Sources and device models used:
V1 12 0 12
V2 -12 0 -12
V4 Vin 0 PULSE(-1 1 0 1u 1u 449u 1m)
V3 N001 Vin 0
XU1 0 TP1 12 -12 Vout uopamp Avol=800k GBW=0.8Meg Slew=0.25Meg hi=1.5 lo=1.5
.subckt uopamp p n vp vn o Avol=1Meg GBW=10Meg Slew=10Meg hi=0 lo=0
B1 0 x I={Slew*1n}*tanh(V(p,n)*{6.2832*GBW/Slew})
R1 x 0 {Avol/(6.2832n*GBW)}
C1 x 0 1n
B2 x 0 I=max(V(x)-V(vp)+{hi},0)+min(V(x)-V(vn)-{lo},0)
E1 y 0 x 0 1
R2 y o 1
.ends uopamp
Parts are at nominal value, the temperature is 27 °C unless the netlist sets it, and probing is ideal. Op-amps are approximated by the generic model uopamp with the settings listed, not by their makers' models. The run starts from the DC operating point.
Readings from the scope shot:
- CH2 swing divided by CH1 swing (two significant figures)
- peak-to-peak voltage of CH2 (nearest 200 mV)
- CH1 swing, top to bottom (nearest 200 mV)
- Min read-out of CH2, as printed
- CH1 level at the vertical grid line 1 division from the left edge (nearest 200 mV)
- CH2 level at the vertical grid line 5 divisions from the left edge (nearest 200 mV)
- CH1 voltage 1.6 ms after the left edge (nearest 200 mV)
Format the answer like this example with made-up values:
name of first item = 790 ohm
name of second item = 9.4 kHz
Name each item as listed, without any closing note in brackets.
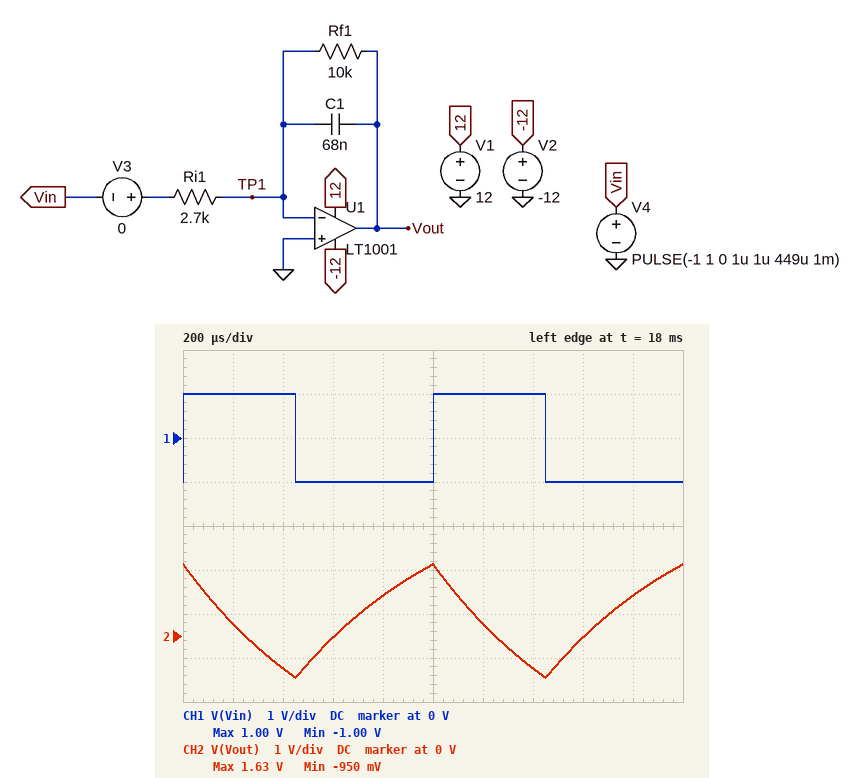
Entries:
CH2 swing divided by CH1 swing = 1.3
peak-to-peak voltage of CH2 = 2.6 V
CH1 swing, top to bottom = 2.0 V
Min read-out of CH2, as printed = -950 mV
CH1 level at the vertical grid line 1 division from the left edge = 1.0 V
CH2 level at the vertical grid line 5 divisions from the left edge = 1.6 V
CH1 voltage 1.6 ms after the left edge = -1.0 V
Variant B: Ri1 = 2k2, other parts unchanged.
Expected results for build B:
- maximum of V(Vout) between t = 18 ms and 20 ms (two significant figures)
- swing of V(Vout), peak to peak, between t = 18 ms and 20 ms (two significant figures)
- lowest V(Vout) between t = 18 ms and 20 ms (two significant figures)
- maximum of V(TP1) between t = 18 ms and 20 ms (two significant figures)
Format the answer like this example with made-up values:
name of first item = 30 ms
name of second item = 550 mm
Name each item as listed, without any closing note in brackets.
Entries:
maximum of V(Vout) between t = 18 ms and 20 ms = 2.0 V
swing of V(Vout), peak to peak, between t = 18 ms and 20 ms = 3.2 V
lowest V(Vout) between t = 18 ms and 20 ms = -1.2 V
maximum of V(TP1) between t = 18 ms and 20 ms = 1.9 mV
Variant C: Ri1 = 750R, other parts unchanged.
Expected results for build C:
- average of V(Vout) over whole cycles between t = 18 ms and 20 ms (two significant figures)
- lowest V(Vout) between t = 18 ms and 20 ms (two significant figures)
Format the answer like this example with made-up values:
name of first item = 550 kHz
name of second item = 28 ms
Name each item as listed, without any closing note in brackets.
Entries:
average of V(Vout) over whole cycles between t = 18 ms and 20 ms = 1.3 V
lowest V(Vout) between t = 18 ms and 20 ms = -3.4 V
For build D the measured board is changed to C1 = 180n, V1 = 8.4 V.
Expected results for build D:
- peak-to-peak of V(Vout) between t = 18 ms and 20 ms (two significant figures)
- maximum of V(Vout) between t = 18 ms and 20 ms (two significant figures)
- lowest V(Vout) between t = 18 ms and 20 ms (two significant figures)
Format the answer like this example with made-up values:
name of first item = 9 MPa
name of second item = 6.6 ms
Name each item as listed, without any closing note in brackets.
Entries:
peak-to-peak of V(Vout) between t = 18 ms and 20 ms = 1.0 V
maximum of V(Vout) between t = 18 ms and 20 ms = 870 mV
lowest V(Vout) between t = 18 ms and 20 ms = -140 mV
